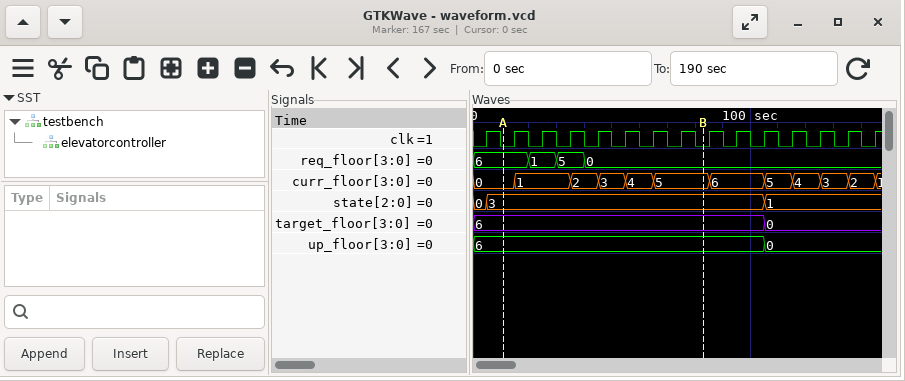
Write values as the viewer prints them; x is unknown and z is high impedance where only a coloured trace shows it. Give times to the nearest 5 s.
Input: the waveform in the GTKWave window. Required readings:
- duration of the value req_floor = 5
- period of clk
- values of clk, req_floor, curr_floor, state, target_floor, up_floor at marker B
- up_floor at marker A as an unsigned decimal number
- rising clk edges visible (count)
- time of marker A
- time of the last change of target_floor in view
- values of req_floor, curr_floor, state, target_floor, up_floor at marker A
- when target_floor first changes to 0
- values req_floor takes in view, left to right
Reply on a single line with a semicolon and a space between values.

10 s; 10 s; clk=0, req_floor=0, curr_floor=5, state=3, target_floor=6, up_floor=6; 6; 15; 10 s; 105 s; req_floor=6, curr_floor=0, state=3, target_floor=6, up_floor=6; 105 s; 6, 1, 5, 0
